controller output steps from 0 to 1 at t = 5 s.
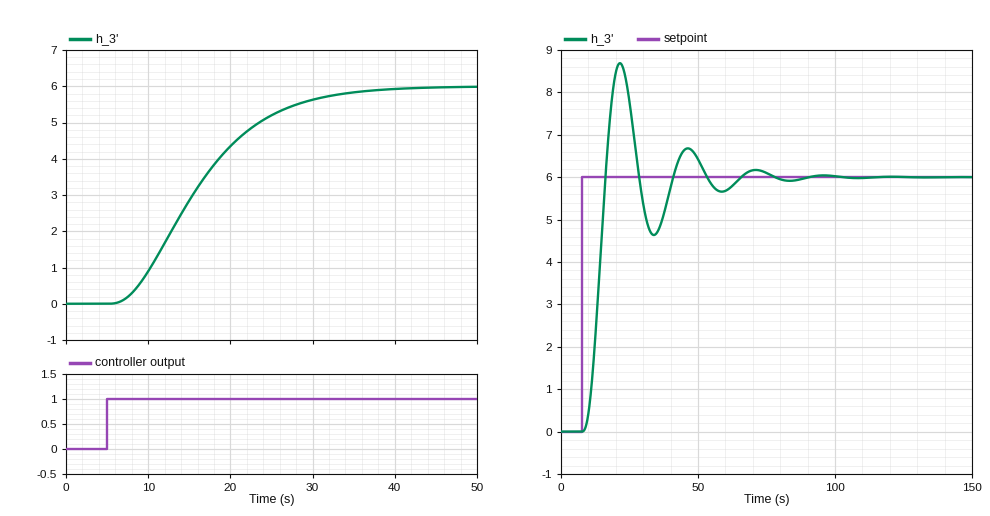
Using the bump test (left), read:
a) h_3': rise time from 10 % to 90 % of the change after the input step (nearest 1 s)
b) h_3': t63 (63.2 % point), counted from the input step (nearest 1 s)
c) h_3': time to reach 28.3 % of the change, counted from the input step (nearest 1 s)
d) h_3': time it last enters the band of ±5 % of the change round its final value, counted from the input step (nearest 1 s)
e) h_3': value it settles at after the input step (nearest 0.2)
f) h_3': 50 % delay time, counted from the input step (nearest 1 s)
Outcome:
18 s
13 s
7 s
26 s
6.0
10 s
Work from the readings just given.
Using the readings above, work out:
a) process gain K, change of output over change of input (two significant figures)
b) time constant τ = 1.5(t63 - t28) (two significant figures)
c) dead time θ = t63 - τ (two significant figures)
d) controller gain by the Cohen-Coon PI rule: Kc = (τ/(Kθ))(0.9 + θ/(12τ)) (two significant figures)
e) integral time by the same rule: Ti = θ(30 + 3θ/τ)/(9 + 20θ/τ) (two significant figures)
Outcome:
6.0
9.0 s
4.0 s
0.35
7.0 s
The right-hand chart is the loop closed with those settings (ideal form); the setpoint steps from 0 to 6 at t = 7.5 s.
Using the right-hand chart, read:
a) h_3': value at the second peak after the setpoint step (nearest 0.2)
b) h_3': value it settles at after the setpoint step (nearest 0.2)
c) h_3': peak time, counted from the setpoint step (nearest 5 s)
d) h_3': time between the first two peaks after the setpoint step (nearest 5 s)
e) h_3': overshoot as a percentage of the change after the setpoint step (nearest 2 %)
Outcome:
6.6
6.0
15 s
25 s
44 %
